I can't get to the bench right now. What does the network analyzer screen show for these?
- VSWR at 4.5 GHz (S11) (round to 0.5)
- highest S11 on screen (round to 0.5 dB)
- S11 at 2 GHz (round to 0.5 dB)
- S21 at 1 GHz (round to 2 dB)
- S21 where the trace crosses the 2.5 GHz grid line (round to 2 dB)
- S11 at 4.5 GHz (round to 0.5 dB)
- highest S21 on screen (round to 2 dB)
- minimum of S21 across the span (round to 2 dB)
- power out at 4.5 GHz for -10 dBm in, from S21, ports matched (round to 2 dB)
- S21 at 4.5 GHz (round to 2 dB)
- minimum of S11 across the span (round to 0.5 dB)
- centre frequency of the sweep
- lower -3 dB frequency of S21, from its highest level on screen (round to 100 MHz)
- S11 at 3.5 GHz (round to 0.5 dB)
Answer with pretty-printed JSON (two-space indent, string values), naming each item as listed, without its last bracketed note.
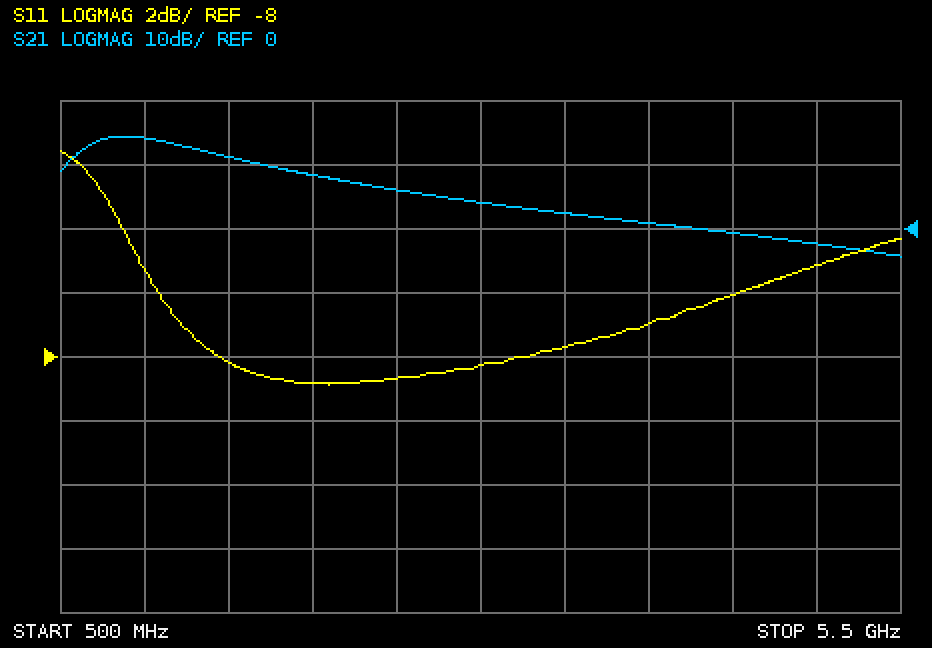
{
  "VSWR at 4.5 GHz (S11)": "3.0",
  "highest S11 on screen": "-1.5 dB",
  "S11 at 2 GHz": "-9.0 dB",
  "S21 at 1 GHz": "14 dB",
  "S21 where the trace crosses the 2.5 GHz grid line": "6 dB",
  "S11 at 4.5 GHz": "-6.0 dB",
  "highest S21 on screen": "14 dB",
  "minimum of S21 across the span": "-4 dB",
  "power out at 4.5 GHz for -10 dBm in, from S21, ports matched": "-10 dBm",
  "S21 at 4.5 GHz": "0 dB",
  "minimum of S11 across the span": "-9.0 dB",
  "centre frequency of the sweep": "3 GHz",
  "lower -3 dB frequency of S21, from its highest level on screen": "600 MHz",
  "S11 at 3.5 GHz": "-7.5 dB"
}
